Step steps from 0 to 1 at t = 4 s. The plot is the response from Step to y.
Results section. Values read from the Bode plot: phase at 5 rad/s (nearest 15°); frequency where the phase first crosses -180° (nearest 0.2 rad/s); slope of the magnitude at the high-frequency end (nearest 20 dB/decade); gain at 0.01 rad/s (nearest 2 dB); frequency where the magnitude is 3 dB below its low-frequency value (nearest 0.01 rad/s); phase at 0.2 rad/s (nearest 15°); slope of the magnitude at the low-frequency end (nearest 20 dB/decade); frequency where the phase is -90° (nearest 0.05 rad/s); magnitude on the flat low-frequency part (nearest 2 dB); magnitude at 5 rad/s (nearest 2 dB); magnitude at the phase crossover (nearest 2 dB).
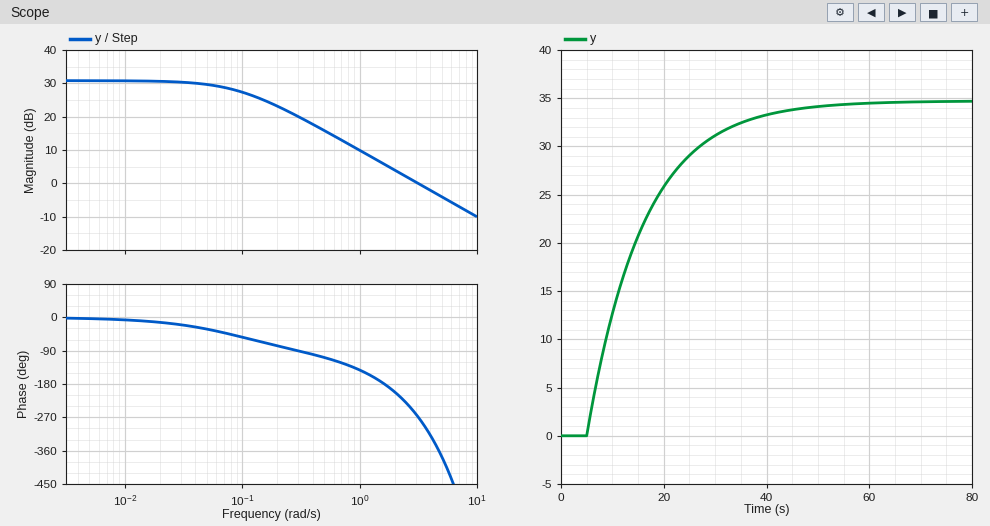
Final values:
-375°
1.6 rad/s
-20 dB/decade
30 dB
0.09 rad/s
-75°
0 dB/decade
0.30 rad/s
30 dB
-4 dB
6 dB
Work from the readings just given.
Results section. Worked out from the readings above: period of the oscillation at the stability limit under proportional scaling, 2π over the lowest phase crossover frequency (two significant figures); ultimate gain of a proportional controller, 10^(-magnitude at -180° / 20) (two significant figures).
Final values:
3.9 s
0.50
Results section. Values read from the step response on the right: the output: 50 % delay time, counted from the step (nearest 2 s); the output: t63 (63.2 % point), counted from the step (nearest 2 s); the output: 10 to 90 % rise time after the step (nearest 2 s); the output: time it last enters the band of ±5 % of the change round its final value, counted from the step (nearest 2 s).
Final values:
8 s
12 s
24 s
34 s
